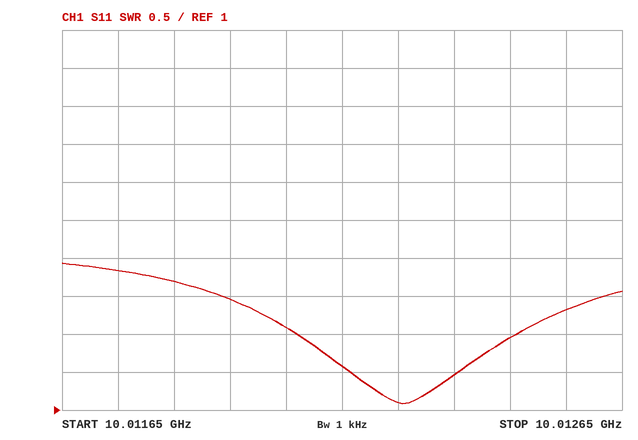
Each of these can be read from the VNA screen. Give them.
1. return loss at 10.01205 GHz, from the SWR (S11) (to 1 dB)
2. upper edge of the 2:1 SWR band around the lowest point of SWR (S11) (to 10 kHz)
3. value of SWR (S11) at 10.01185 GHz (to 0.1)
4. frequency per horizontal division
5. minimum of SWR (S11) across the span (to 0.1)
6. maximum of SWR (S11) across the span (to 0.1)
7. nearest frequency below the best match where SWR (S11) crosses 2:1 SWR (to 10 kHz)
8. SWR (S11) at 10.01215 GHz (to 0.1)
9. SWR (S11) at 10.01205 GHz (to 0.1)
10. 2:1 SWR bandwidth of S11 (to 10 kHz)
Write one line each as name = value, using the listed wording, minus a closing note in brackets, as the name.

return loss at 10.01205 GHz, from the SWR (S11) = 9 dB
upper edge of the 2:1 SWR band around the lowest point of SWR (S11) = 10.01246 GHz
value of SWR (S11) at 10.01185 GHz = 2.7
frequency per horizontal division = 100 kHz
minimum of SWR (S11) across the span = 1.1
maximum of SWR (S11) across the span = 2.9
nearest frequency below the best match where SWR (S11) crosses 2:1 SWR = 10.01207 GHz
SWR (S11) at 10.01215 GHz = 1.6
SWR (S11) at 10.01205 GHz = 2.1
2:1 SWR bandwidth of S11 = 390 kHz
